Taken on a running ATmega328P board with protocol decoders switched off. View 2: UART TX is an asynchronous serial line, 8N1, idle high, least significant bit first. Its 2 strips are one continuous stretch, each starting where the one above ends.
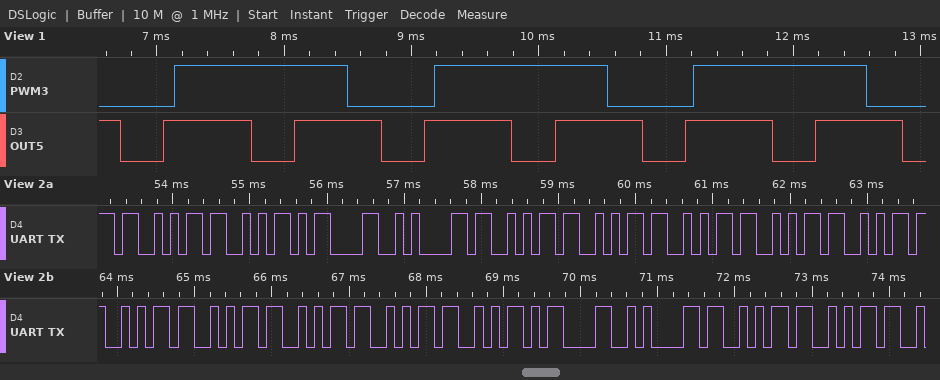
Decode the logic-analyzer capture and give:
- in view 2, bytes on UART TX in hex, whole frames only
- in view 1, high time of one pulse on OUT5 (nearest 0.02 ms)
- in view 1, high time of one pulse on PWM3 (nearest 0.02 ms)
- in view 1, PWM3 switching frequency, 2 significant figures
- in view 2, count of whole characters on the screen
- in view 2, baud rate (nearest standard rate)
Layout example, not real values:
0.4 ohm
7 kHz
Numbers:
53 53 0D 0A 53 53 53 53 53 53 53 53 53 53 0D 0A 53 53
0.68 ms
1.36 ms
490 Hz
18
9600 baud
